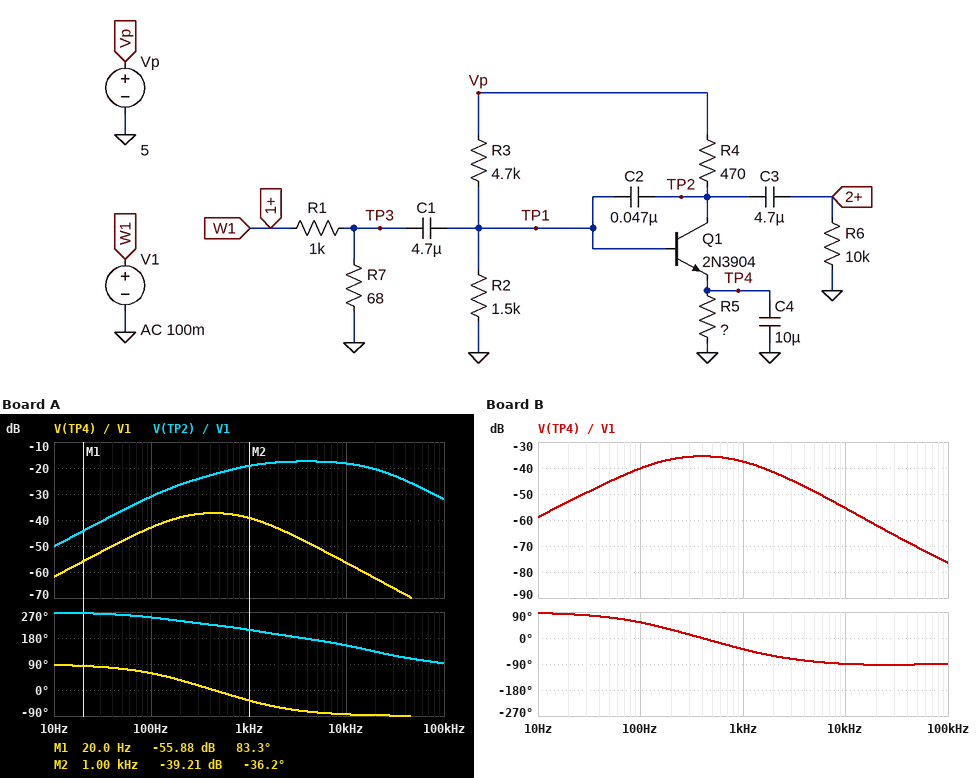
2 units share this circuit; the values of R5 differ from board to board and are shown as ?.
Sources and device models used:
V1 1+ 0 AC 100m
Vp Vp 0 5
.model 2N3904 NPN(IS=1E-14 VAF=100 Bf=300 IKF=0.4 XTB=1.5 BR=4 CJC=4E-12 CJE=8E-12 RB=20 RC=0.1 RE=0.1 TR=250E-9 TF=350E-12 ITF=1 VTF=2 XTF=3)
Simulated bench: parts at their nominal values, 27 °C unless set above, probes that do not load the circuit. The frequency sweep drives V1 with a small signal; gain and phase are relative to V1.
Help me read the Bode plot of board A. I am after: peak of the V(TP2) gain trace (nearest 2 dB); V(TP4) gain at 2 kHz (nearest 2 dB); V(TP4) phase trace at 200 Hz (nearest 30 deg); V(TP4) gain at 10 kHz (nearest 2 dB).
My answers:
-18 dB
-44 dB
30 deg
-56 dB
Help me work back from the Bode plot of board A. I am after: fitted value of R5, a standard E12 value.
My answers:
33 Ω
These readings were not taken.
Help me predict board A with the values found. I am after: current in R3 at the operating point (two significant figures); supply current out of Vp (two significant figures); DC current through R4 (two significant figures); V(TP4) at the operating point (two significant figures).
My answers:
840 µA
11 mA
9.8 mA
330 mV
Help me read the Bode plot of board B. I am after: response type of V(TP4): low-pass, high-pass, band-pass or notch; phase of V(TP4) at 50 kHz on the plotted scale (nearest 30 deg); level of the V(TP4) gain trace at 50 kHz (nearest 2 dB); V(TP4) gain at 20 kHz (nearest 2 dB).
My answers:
band-pass
-90 deg
-70 dB
-62 dB
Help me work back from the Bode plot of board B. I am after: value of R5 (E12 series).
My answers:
39 Ω
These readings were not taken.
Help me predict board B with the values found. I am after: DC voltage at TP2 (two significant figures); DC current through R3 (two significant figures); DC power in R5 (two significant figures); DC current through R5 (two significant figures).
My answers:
480 mV
830 µA
3.7 mW
9.7 mA
